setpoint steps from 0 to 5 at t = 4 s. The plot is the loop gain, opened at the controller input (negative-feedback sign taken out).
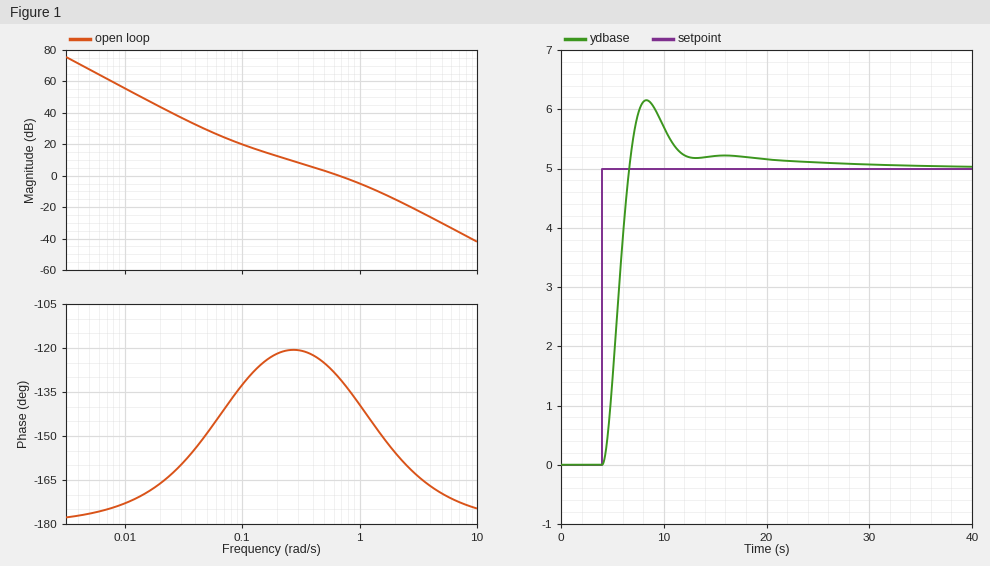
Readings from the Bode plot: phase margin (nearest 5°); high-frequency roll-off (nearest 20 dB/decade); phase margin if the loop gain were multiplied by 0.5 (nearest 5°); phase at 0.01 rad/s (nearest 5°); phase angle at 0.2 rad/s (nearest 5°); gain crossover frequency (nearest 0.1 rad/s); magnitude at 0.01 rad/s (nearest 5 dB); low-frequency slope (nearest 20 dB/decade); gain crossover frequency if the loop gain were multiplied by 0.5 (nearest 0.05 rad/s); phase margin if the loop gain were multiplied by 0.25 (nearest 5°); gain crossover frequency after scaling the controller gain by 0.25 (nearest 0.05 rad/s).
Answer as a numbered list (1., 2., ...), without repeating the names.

1. 50°
2. -40 dB/decade
3. 60°
4. -175°
5. -120°
6. 0.7 rad/s
7. 55 dB
8. -40 dB/decade
9. 0.40 rad/s
10. 60°
11. 0.20 rad/s
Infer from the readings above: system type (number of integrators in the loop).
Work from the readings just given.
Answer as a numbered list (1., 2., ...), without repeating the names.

1. 2
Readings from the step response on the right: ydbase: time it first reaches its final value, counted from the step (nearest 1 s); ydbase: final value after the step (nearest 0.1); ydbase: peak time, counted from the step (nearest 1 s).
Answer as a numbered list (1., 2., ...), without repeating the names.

1. 3 s
2. 5.0
3. 4 s
